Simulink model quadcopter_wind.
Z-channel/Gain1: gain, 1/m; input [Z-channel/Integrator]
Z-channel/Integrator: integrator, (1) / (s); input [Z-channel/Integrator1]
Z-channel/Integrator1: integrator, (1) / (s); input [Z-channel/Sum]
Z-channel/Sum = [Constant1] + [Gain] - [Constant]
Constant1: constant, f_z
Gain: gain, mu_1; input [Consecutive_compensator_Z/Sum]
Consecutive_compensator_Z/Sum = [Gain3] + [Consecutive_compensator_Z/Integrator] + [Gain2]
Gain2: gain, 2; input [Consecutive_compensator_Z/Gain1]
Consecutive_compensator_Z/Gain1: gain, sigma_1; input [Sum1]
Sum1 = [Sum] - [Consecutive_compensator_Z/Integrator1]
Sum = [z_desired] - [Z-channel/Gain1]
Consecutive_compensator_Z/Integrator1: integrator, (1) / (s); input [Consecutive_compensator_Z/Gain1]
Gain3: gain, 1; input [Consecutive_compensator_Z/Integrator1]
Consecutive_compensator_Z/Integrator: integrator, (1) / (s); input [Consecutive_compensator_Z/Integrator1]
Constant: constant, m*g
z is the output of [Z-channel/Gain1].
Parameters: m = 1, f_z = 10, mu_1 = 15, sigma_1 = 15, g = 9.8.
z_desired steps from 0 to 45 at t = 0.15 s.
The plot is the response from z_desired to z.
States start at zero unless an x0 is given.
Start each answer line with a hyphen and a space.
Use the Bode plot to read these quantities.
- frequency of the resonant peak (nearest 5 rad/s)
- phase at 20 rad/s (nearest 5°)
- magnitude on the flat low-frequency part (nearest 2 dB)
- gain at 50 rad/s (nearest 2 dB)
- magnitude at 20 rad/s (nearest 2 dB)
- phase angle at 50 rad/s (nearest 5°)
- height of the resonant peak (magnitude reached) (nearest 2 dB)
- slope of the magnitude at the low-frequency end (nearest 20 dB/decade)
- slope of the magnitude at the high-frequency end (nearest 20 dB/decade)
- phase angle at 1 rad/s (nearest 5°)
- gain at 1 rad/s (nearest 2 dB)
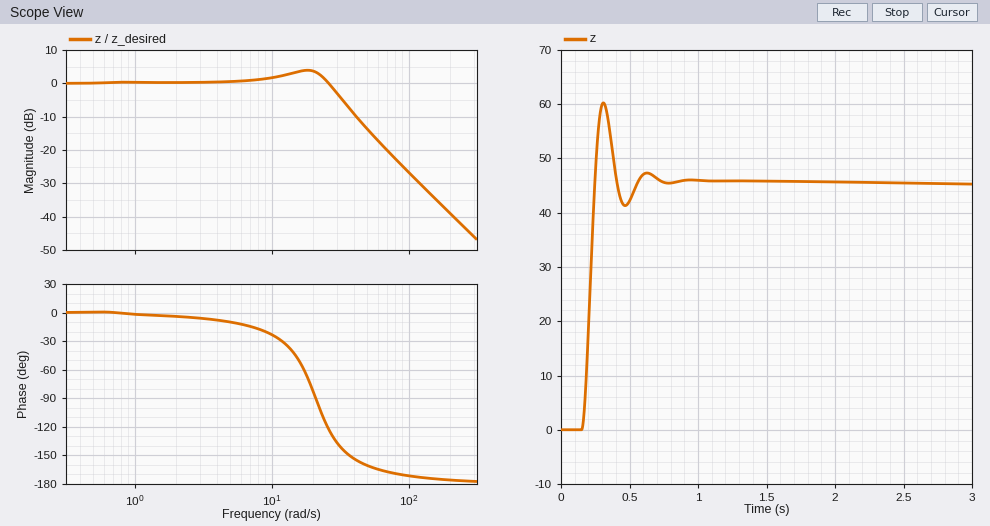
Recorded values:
- 20 rad/s
- -80°
- 0 dB
- -14 dB
- 4 dB
- -160°
- 4 dB
- 0 dB/decade
- -40 dB/decade
- 0°
- 0 dB
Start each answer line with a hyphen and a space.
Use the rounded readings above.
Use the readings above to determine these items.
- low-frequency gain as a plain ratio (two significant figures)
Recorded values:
- 1.0
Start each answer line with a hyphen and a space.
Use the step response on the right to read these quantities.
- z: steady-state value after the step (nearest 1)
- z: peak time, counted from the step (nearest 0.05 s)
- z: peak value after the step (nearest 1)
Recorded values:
- 45
- 0.15 s
- 60
